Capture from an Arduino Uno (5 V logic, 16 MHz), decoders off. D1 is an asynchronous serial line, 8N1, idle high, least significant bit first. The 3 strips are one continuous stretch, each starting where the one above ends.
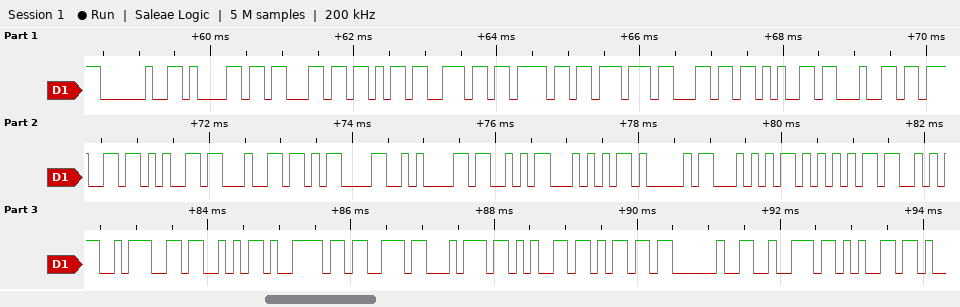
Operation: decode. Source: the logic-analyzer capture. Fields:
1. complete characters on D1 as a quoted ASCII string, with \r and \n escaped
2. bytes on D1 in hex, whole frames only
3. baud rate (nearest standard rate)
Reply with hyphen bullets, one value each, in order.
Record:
- " acknowledged\r\nSTATUS:System re"
- 20 61 63 6B 6E 6F 77 6C 65 64 67 65 64 0D 0A 53 54 41 54 55 53 3A 53 79 73 74 65 6D 20 72 65
- 9600 baud
